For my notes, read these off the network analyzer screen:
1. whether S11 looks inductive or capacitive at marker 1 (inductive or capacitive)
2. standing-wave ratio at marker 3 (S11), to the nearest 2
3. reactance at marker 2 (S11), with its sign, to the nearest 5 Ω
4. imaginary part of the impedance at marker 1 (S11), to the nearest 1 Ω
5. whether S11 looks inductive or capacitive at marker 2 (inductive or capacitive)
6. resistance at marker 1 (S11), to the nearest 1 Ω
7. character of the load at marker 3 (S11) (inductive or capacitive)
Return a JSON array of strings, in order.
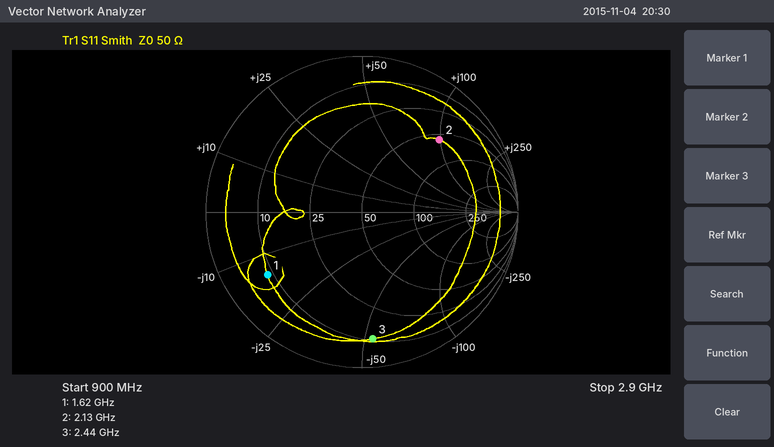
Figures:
["capacitive", "10", "+100 Ω", "-15 Ω", "inductive", "9 Ω", "capacitive"]
